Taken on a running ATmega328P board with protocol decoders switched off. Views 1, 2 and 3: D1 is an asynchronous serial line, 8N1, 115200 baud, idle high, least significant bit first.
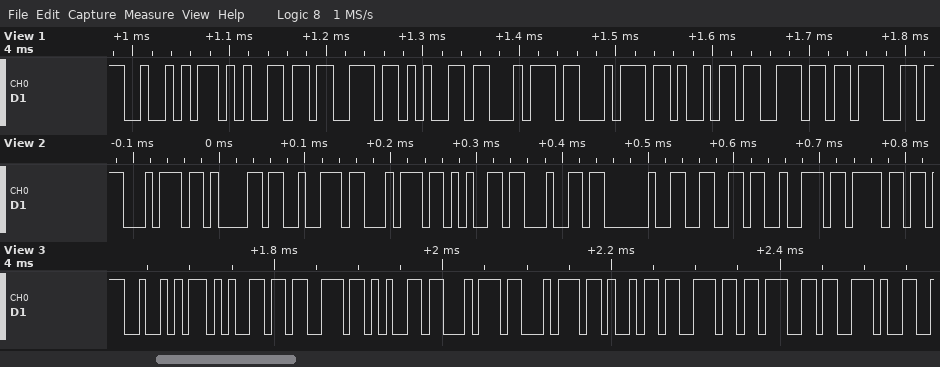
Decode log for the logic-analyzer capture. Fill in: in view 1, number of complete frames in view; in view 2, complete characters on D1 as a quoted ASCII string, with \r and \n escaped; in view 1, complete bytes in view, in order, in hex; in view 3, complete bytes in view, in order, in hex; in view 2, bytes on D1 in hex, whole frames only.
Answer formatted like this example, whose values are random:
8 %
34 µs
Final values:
9
"tarted fro"
52 65 73 65 74 74 69 6E 67
52 65 73 65 74 74 69 6E 67 2E
0x74 0x61 0x72 0x74 0x65 0x64 0x20 0x66 0x72 0x6F
